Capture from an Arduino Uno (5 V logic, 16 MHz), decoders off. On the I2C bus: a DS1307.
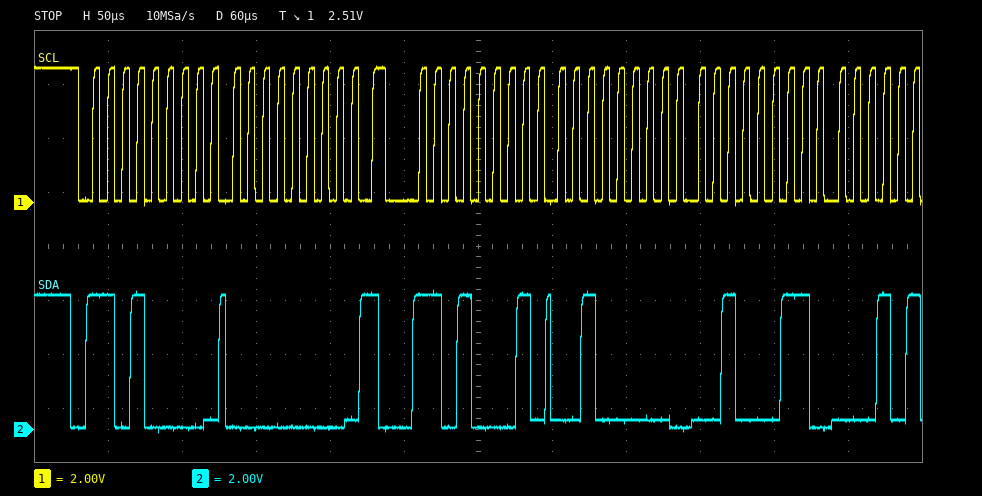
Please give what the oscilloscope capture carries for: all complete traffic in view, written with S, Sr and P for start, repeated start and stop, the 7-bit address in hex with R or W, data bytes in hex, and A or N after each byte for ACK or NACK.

S 68W A 00 A Sr 68R A 20 A 23 A
